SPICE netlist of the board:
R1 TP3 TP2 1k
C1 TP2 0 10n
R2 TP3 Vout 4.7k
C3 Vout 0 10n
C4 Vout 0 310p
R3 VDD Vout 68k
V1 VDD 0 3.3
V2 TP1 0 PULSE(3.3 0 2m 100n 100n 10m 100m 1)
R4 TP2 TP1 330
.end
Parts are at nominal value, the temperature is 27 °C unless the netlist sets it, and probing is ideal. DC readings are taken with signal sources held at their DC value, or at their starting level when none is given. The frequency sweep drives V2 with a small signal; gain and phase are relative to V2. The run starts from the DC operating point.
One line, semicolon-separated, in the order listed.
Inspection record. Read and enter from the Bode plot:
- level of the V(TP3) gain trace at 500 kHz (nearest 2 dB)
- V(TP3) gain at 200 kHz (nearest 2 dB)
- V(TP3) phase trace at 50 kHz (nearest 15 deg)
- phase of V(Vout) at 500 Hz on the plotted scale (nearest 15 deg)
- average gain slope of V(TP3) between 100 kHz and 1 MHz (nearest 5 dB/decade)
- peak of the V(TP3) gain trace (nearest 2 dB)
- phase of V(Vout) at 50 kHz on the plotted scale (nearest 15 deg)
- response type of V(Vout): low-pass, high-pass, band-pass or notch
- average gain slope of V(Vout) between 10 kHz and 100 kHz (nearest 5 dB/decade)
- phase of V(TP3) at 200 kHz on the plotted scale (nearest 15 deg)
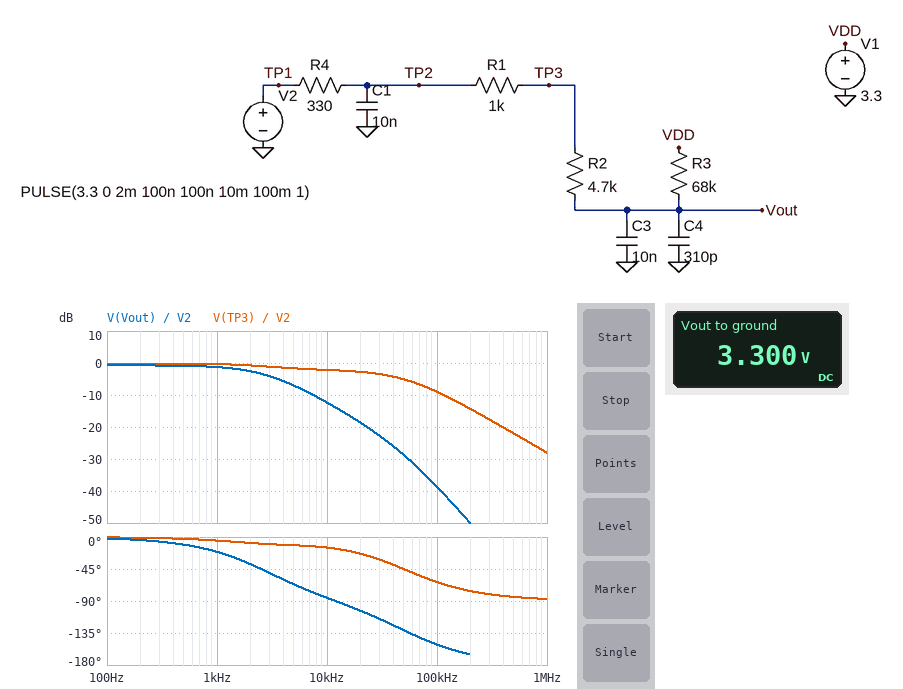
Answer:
-22 dB; -14 dB; -45 deg; -15 deg; -20 dB/decade; 0 dB; -135 deg; low-pass; -25 dB/decade; -75 deg
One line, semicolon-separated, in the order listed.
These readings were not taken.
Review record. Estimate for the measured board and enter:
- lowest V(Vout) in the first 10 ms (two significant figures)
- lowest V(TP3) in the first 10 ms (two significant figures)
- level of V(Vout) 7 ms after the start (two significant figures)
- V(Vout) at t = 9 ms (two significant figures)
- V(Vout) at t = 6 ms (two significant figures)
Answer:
270 mV; 59 mV; 270 mV; 270 mV; 270 mV
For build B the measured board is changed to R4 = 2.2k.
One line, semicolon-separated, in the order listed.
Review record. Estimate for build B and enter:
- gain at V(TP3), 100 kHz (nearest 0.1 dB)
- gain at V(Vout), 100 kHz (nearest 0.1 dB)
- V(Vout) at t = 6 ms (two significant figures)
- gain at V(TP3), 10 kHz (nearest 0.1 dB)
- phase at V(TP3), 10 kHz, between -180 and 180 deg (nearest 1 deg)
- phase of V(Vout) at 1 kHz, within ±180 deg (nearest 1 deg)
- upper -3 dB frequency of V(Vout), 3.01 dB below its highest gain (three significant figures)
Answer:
-24.5 dB; -54.2 dB; 340 mV; -7.6 dB; -50 deg; -32 deg; 1.93 kHz
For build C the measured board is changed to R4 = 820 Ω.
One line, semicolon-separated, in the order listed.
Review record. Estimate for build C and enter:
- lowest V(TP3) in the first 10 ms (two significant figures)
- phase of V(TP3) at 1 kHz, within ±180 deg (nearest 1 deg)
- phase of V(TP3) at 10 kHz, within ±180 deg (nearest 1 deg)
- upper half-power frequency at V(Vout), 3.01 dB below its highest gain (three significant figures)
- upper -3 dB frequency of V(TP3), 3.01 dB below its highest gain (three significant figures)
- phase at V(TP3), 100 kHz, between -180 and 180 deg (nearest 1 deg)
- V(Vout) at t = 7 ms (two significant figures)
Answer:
81 mV; -8 deg; -29 deg; 2.52 kHz; 8.33 kHz; -78 deg; 290 mV
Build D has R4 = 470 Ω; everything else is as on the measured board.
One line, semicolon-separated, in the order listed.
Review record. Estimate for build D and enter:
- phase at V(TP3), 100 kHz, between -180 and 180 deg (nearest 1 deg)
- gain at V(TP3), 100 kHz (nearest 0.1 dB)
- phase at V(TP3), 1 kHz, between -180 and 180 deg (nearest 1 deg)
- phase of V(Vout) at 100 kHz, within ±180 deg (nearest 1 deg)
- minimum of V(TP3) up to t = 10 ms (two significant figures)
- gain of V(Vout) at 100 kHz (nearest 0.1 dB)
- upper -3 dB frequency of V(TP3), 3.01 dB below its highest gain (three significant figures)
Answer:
-70 deg; -11.6 dB; -6 deg; -158 deg; 65 mV; -41.3 dB; 17.0 kHz
